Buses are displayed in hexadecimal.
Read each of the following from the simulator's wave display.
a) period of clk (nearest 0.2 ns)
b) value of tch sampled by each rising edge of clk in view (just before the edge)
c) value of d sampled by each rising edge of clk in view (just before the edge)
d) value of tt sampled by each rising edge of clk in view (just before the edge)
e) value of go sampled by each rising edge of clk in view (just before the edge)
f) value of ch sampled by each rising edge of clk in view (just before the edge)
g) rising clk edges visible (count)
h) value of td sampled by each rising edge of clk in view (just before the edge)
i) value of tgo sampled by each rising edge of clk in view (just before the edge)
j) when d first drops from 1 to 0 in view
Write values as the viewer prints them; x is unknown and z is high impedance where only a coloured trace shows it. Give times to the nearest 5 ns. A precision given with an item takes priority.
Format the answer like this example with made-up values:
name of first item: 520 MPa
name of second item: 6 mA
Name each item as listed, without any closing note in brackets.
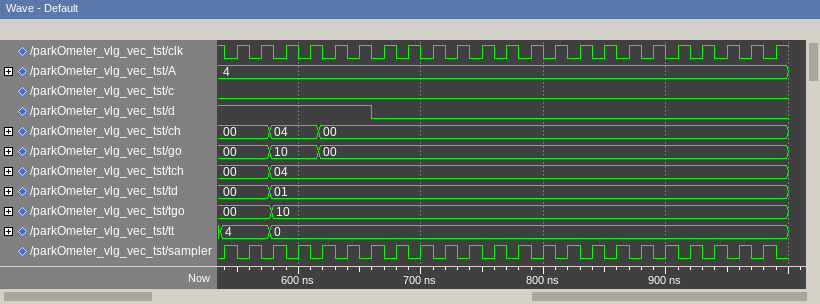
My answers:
period of clk: 20 ns
value of tch sampled by each rising edge of clk in view: 00, 00, 04, 04, 04, 04, 04, 04, 04, 04, 04, 04, 04, 04, 04, 04, 04, 04, 04, 04, 04, 04, 04
value of d sampled by each rising edge of clk in view: 1 1 1 1 1 1 0 0 0 0 0 0 0 0 0 0 0 0 0 0 0 0 0
value of tt sampled by each rising edge of clk in view: 4, 4, 0, 0, 0, 0, 0, 0, 0, 0, 0, 0, 0, 0, 0, 0, 0, 0, 0, 0, 0, 0, 0
value of go sampled by each rising edge of clk in view: 00, 00, 10, 10, 00, 00, 00, 00, 00, 00, 00, 00, 00, 00, 00, 00, 00, 00, 00, 00, 00, 00, 00
value of ch sampled by each rising edge of clk in view: 00, 00, 04, 04, 00, 00, 00, 00, 00, 00, 00, 00, 00, 00, 00, 00, 00, 00, 00, 00, 00, 00, 00
rising clk edges visible: 23
value of td sampled by each rising edge of clk in view: 00, 00, 01, 01, 01, 01, 01, 01, 01, 01, 01, 01, 01, 01, 01, 01, 01, 01, 01, 01, 01, 01, 01
value of tgo sampled by each rising edge of clk in view: 00, 00, 10, 10, 10, 10, 10, 10, 10, 10, 10, 10, 10, 10, 10, 10, 10, 10, 10, 10, 10, 10, 10
when d first drops from 1 to 0 in view: 660 ns
